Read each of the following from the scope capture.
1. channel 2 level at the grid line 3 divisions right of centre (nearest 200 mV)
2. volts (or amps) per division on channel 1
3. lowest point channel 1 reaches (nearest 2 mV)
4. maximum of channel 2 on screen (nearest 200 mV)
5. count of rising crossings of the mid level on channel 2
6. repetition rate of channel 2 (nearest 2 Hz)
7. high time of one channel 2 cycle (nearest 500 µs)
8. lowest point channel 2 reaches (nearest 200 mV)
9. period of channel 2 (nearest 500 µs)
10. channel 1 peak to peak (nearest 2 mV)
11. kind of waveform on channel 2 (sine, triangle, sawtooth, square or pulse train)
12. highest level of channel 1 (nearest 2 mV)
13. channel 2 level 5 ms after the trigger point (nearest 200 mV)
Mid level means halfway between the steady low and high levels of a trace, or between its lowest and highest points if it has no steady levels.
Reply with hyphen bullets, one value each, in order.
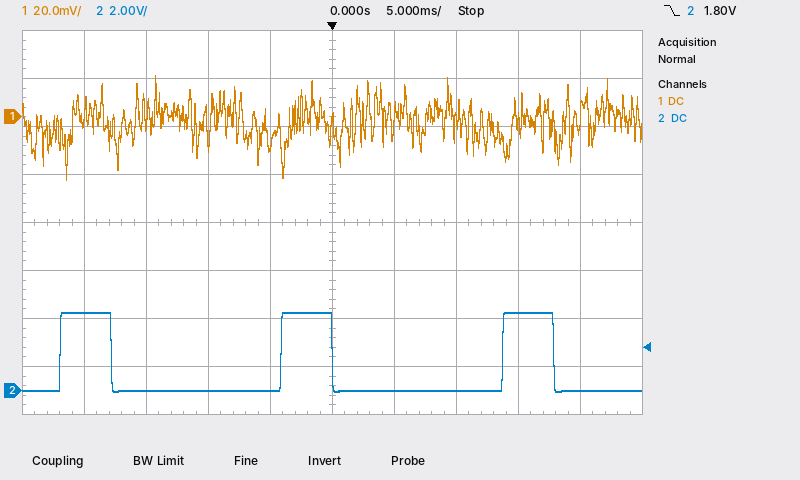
- 3.2 V
- 20 mV
- -26 mV
- 3.2 V
- 3
- 56 Hz
- 4.0 ms
- 0.0 V
- 18.0 ms
- 44 mV
- pulse train
- 18 mV
- 0.0 V
